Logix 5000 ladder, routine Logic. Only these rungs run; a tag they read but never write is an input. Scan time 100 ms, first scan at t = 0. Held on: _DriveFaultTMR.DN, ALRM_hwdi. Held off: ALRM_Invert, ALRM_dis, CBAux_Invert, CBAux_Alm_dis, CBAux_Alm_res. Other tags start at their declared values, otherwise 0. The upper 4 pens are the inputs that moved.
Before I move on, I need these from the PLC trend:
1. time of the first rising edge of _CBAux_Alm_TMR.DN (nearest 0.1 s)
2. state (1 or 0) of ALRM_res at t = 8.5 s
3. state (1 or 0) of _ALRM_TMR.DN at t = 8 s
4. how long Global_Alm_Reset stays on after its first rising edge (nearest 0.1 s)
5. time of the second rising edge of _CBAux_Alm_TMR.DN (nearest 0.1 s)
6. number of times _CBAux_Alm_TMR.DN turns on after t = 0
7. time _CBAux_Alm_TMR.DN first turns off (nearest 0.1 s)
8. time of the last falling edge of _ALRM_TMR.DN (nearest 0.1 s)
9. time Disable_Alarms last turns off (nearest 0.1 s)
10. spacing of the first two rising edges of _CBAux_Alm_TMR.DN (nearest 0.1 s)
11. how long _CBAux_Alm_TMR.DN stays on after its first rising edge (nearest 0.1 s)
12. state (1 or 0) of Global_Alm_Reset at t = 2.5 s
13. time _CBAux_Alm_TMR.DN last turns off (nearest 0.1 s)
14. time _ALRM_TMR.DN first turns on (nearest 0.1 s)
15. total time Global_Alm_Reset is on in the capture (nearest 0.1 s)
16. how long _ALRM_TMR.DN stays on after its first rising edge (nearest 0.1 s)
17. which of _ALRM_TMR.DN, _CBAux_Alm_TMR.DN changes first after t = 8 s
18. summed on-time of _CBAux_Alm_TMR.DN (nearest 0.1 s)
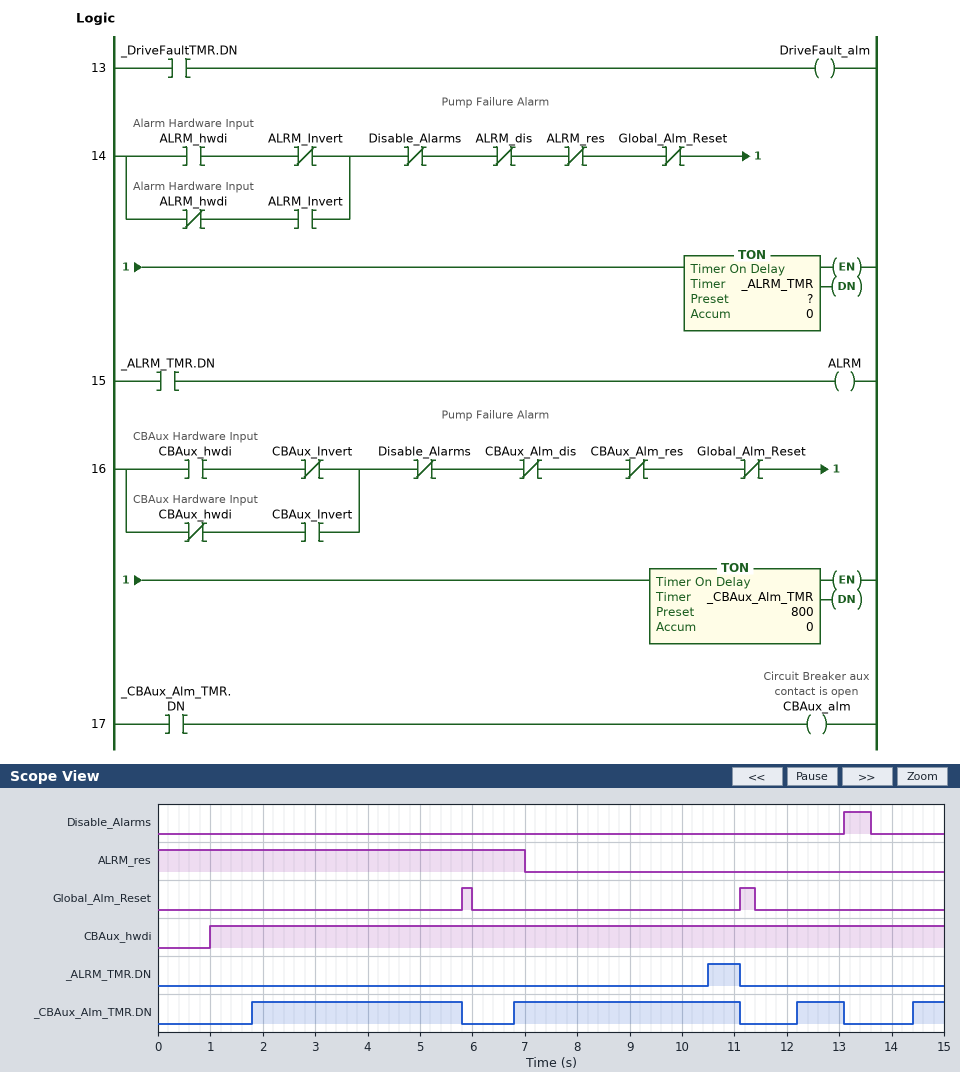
1.8 s
0
0
0.2 s
6.8 s
4
5.8 s
11.1 s
13.6 s
5.0 s
4.0 s
0
13.1 s
10.5 s
0.5 s
0.6 s
_ALRM_TMR.DN
9.8 s
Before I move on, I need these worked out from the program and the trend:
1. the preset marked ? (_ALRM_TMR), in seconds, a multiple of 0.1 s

3.5 s
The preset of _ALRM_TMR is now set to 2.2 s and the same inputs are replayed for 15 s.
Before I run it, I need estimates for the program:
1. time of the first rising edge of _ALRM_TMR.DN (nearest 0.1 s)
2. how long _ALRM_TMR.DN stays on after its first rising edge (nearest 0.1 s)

9.2 s
1.9 s
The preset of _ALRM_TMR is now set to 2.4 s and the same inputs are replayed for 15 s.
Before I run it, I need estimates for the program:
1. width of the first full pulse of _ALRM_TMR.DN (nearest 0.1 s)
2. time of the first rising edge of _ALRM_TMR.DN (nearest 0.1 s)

1.7 s
9.4 s
